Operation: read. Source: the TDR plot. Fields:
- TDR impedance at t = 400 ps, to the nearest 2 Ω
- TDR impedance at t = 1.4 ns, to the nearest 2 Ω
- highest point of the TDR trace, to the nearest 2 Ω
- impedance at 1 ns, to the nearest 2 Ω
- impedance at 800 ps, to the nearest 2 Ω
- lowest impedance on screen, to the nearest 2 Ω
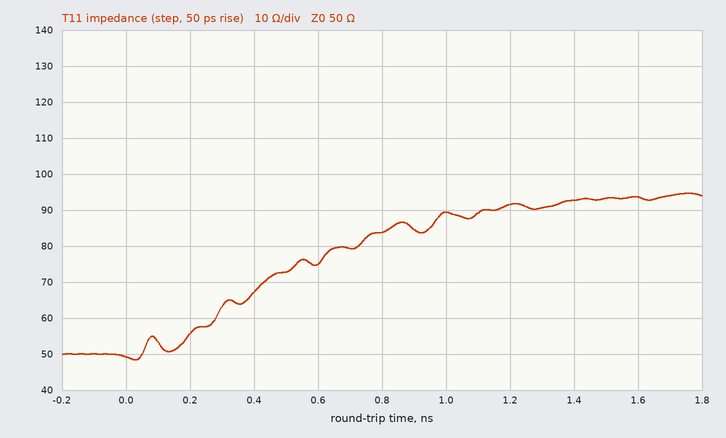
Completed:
68 Ω
92 Ω
94 Ω
90 Ω
84 Ω
48 Ω
